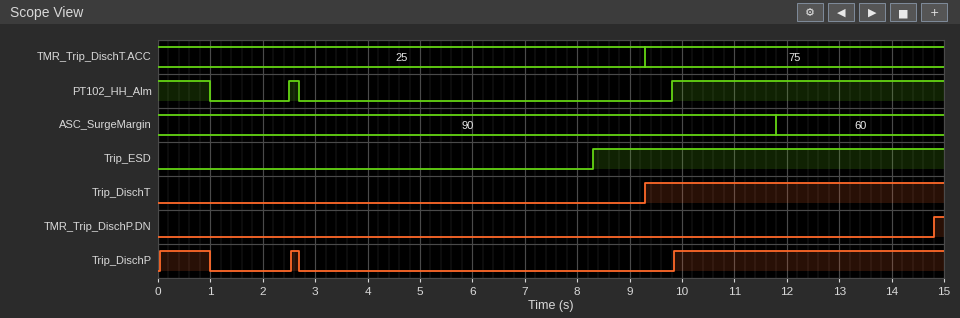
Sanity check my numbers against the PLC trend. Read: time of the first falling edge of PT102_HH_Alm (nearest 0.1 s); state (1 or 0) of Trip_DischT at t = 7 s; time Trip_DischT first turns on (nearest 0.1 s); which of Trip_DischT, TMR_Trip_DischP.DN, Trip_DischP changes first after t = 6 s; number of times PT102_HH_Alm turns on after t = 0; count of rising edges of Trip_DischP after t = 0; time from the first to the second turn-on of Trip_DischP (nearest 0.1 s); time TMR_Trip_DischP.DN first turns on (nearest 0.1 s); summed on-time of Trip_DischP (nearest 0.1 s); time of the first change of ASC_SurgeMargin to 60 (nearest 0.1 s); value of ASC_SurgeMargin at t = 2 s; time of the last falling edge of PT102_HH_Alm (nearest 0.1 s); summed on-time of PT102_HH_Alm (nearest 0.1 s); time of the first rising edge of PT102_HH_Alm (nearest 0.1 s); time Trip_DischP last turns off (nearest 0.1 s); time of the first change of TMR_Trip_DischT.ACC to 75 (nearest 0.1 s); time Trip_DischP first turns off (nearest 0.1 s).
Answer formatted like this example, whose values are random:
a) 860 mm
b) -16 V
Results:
a) 1.0 s
b) 0
c) 9.3 s
d) Trip_DischT
e) 2
f) 3
g) 2.5 s
h) 14.8 s
i) 6.3 s
j) 11.8 s
k) 90
l) 2.7 s
m) 6.4 s
n) 2.5 s
o) 2.7 s
p) 9.3 s
q) 1.0 s
